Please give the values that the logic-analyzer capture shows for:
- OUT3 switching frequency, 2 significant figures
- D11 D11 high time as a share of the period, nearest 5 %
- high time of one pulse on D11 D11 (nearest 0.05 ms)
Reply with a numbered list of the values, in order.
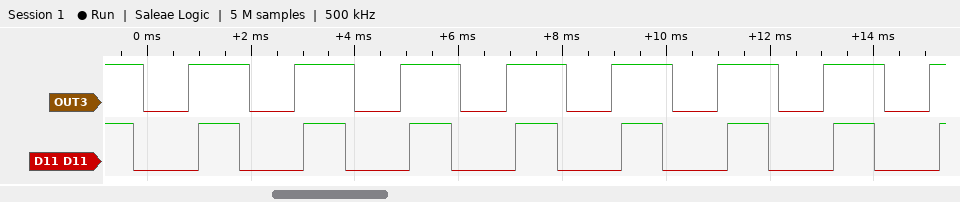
1. 490 Hz
2. 40 %
3. 0.80 ms
